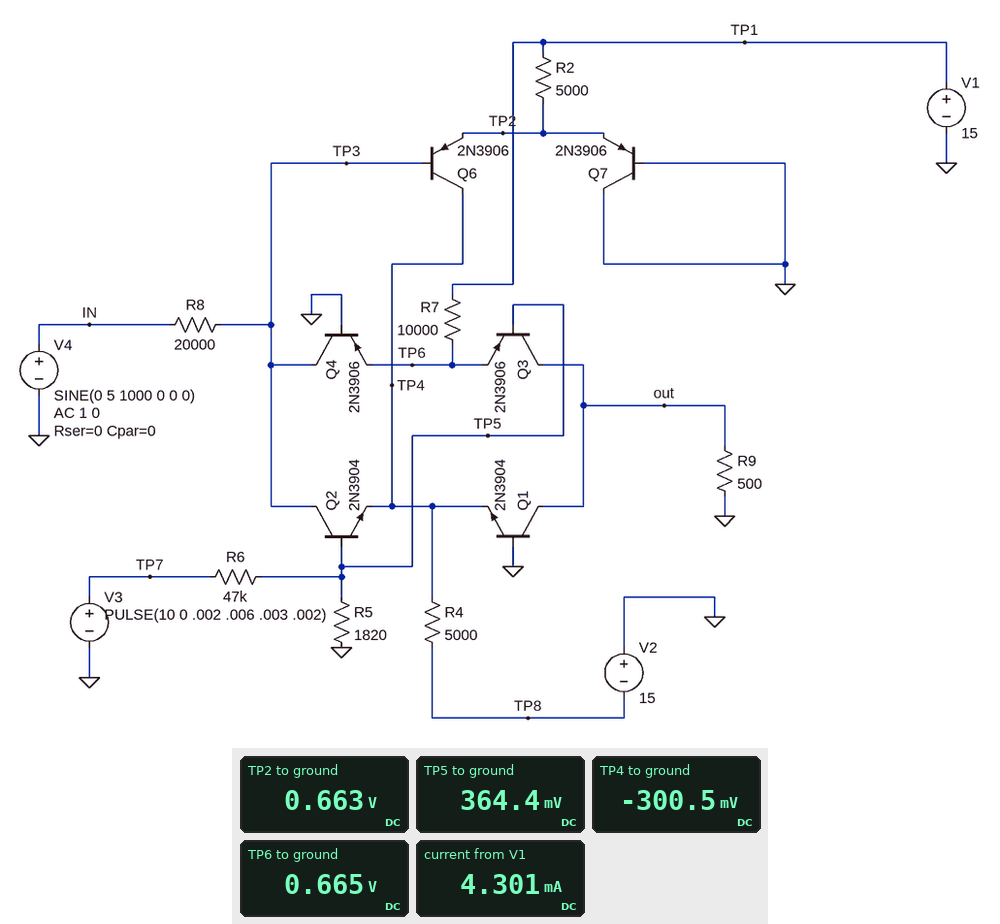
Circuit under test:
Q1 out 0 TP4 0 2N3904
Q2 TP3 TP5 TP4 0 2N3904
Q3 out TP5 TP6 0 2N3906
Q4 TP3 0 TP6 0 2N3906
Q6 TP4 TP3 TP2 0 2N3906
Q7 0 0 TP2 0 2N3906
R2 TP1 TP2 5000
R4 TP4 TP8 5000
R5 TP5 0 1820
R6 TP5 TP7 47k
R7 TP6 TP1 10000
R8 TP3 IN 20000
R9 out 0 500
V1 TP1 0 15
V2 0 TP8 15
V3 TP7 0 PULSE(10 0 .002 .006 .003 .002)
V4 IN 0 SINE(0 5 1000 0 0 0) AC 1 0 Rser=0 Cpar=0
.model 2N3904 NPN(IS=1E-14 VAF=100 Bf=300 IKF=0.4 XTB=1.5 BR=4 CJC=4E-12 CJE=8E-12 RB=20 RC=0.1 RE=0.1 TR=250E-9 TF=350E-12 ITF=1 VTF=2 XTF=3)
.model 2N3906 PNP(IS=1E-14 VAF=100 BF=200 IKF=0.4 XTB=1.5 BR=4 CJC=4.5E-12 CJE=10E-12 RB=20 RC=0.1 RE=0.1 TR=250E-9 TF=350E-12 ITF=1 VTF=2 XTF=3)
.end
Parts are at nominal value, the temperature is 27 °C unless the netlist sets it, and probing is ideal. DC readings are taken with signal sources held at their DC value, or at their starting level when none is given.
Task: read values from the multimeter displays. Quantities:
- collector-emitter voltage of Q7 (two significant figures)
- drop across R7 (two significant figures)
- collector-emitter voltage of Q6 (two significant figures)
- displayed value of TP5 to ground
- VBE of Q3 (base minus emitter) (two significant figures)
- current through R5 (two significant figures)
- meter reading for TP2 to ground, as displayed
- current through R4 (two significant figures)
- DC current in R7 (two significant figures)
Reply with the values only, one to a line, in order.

-660 mV
14 V
-960 mV
364.4 mV
-300 mV
200 µA
0.663 V
2.9 mA
1.4 mA
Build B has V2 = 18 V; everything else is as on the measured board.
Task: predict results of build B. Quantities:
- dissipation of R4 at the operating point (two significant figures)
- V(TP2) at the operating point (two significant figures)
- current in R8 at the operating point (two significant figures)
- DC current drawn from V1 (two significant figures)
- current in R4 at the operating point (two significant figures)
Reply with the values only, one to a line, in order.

63 mW
650 mV
1.3 µA
4.3 mA
3.5 mA
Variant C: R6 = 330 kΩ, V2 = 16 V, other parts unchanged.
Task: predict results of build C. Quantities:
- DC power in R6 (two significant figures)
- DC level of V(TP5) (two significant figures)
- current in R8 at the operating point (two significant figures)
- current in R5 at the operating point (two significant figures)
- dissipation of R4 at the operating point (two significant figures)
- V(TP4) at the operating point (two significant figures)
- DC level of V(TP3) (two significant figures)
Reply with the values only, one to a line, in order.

300 µW
49 mV
380 nA
27 µA
47 mW
-610 mV
-7.6 mV
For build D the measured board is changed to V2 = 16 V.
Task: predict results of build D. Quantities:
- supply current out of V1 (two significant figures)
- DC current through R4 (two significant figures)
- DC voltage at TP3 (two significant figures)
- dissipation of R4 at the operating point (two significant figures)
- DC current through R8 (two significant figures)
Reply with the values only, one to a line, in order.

4.3 mA
3.1 mA
-10 mV
49 mW
500 nA
